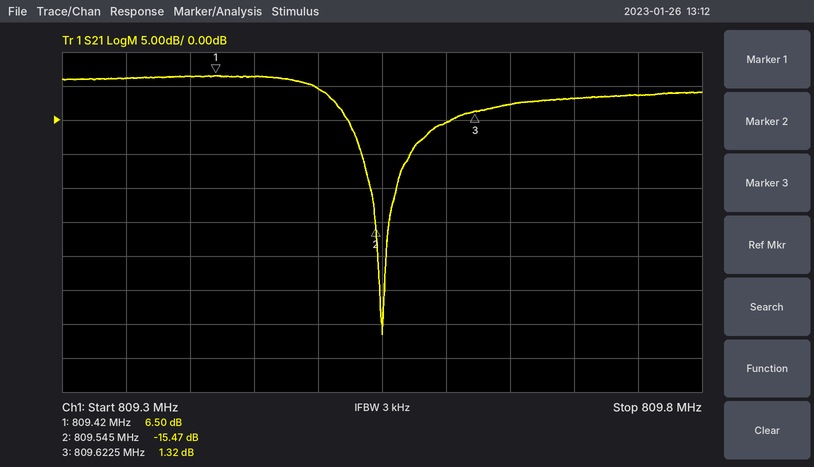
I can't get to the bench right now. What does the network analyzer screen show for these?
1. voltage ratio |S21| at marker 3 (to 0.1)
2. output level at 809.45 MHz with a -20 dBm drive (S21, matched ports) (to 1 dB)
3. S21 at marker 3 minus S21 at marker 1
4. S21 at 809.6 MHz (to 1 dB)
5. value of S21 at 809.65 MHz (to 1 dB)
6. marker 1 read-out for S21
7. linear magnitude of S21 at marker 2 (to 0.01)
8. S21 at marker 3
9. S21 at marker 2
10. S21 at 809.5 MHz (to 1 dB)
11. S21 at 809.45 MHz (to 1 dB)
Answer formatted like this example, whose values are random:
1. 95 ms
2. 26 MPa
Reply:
1. 1.2
2. -14 dBm
3. -5.18 dB
4. 0 dB
5. 2 dB
6. 6.50 dB
7. 0.17
8. 1.32 dB
9. -15.47 dB
10. 5 dB
11. 6 dB
